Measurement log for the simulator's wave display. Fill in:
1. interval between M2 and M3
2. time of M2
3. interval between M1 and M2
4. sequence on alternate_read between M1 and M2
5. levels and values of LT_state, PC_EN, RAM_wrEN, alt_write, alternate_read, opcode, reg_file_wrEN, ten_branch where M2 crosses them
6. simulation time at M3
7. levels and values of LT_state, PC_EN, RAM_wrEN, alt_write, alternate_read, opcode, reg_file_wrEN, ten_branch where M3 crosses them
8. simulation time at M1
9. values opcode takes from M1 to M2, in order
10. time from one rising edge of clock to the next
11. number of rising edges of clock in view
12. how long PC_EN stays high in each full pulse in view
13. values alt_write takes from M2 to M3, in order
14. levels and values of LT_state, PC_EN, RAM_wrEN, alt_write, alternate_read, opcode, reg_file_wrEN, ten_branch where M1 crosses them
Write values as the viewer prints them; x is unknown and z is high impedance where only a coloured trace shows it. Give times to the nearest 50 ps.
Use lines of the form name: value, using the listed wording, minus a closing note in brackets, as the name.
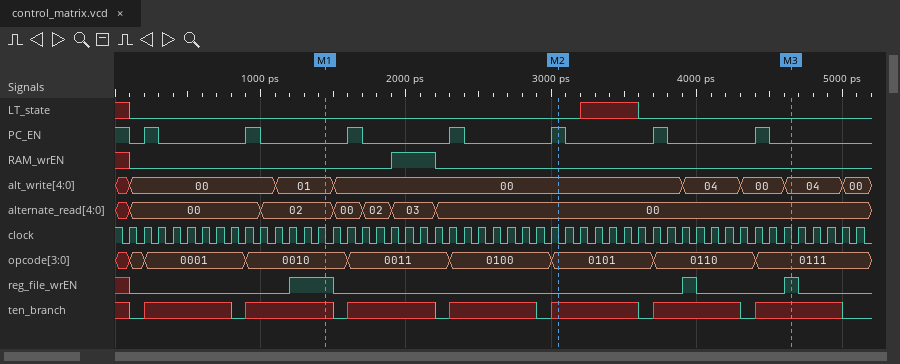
interval between M2 and M3: 1600 ps
time of M2: 3050 ps
interval between M1 and M2: 1600 ps
sequence on alternate_read between M1 and M2: 02, 00, 02, 03, 00
levels and values of LT_state, PC_EN, RAM_wrEN, alt_write, alternate_read, opcode, reg_file_wrEN, ten_branch where M2 crosses them: LT_state=0, PC_EN=1, RAM_wrEN=0, alt_write=00, alternate_read=00, opcode=0101, reg_file_wrEN=0, ten_branch=x
simulation time at M3: 4650 ps
levels and values of LT_state, PC_EN, RAM_wrEN, alt_write, alternate_read, opcode, reg_file_wrEN, ten_branch where M3 crosses them: LT_state=0, PC_EN=0, RAM_wrEN=0, alt_write=04, alternate_read=00, opcode=0111, reg_file_wrEN=1, ten_branch=x
simulation time at M1: 1450 ps
values opcode takes from M1 to M2, in order: 0010, 0011, 0100, 0101
time from one rising edge of clock to the next: 100 ps
number of rising edges of clock in view: 51
how long PC_EN stays high in each full pulse in view: 100 ps, 100 ps, 100 ps, 100 ps, 100 ps, 100 ps, 100 ps
values alt_write takes from M2 to M3, in order: 00, 04, 00, 04
levels and values of LT_state, PC_EN, RAM_wrEN, alt_write, alternate_read, opcode, reg_file_wrEN, ten_branch where M1 crosses them: LT_state=0, PC_EN=0, RAM_wrEN=0, alt_write=01, alternate_read=02, opcode=0010, reg_file_wrEN=1, ten_branch=x
